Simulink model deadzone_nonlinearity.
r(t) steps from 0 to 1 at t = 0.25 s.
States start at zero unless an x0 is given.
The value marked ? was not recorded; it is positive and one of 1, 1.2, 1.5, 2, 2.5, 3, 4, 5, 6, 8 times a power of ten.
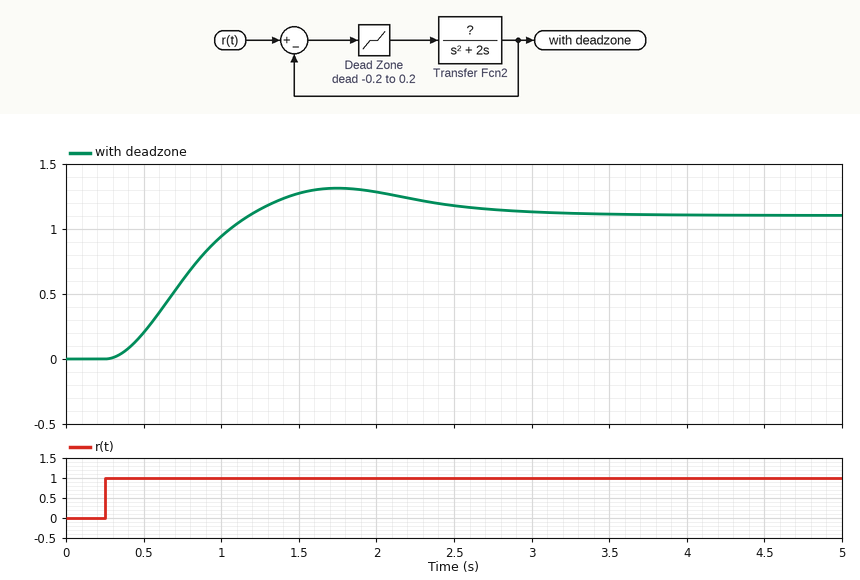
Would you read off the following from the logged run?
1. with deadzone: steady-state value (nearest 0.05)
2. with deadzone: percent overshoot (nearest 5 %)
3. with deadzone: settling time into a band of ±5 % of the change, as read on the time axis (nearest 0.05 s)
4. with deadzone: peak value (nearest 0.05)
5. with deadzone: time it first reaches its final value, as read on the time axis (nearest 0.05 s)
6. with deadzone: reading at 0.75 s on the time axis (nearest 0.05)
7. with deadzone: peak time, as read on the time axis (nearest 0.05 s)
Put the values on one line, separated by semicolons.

1.10; 20 %; 2.65 s; 1.30; 1.20 s; 0.60; 1.75 s
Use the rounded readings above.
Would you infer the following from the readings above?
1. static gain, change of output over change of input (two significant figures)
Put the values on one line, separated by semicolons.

1.1
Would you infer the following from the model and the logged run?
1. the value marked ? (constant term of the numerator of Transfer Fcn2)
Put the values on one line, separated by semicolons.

10
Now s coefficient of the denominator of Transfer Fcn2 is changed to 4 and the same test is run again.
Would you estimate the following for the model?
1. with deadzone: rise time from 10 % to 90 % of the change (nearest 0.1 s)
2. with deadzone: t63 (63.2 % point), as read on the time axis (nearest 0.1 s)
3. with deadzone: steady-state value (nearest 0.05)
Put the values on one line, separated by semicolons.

0.8 s; 0.8 s; 0.90
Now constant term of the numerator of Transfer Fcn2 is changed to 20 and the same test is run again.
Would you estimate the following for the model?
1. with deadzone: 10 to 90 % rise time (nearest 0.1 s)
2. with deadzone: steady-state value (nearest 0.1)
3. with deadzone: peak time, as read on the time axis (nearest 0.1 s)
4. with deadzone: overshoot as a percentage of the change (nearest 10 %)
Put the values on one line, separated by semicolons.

0.3 s; 0.8; 1.2 s; 80 %
